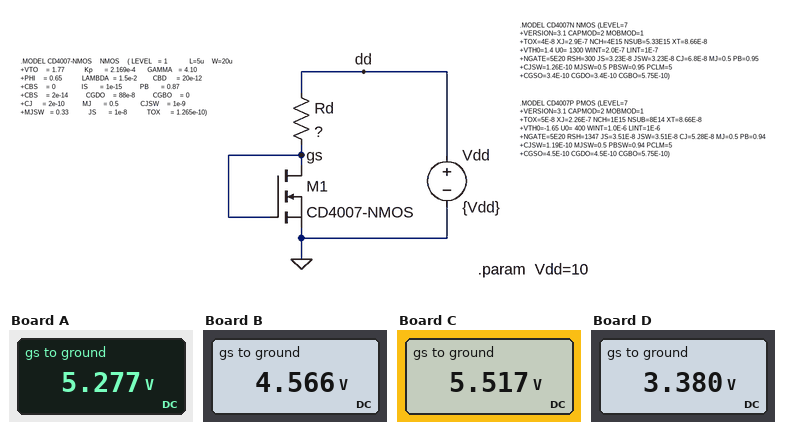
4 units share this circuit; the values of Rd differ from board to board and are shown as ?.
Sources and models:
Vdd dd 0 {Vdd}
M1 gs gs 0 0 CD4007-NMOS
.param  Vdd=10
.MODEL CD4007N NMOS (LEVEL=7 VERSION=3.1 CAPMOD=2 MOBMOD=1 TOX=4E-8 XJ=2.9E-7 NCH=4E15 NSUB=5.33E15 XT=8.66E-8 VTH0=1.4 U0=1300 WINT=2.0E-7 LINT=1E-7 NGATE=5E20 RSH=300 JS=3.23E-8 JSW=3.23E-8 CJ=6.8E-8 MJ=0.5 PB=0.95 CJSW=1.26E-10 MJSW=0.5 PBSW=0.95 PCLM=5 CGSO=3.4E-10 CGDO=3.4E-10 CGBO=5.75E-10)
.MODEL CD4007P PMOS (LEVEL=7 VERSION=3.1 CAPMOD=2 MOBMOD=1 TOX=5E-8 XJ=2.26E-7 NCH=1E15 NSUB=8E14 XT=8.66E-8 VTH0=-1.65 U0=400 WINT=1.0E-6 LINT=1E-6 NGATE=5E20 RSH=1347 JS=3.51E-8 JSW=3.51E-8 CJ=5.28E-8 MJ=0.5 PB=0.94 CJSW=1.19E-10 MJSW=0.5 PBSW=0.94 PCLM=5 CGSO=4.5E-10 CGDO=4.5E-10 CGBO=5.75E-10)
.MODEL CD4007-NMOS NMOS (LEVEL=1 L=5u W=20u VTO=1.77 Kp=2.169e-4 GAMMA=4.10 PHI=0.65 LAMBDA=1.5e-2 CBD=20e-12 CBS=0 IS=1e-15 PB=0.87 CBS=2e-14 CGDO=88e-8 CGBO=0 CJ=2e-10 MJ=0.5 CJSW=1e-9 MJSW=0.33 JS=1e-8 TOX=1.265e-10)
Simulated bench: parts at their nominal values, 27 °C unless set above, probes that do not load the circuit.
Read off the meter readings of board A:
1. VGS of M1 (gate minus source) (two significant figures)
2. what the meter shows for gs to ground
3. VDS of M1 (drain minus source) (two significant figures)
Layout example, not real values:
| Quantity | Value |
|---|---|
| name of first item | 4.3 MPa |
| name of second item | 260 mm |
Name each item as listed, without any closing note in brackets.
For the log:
| Quantity | Value |
|---|---|
| VGS of M1 (gate minus source) | 5.3 V |
| what the meter shows for gs to ground | 5.277 V |
| VDS of M1 (drain minus source) | 5.3 V |
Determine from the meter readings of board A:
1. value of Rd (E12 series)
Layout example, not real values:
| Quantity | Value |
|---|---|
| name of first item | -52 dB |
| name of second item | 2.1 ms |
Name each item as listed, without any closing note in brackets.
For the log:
| Quantity | Value |
|---|---|
| value of Rd | 820 Ω |
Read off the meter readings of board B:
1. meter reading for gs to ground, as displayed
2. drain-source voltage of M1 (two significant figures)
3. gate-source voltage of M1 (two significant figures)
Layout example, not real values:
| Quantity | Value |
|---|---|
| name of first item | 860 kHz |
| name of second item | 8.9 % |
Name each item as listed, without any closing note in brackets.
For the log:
| Quantity | Value |
|---|---|
| meter reading for gs to ground, as displayed | 4.566 V |
| drain-source voltage of M1 | 4.6 V |
| gate-source voltage of M1 | 4.6 V |
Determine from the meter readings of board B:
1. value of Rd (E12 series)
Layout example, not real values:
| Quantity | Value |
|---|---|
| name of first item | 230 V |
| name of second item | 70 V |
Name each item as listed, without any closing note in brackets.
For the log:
| Quantity | Value |
|---|---|
| value of Rd | 1.5 kΩ |
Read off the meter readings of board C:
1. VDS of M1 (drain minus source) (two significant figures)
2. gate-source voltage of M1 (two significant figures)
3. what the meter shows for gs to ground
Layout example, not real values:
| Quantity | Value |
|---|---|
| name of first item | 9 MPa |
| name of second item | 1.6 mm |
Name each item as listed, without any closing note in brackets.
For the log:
| Quantity | Value |
|---|---|
| VDS of M1 (drain minus source) | 5.5 V |
| gate-source voltage of M1 | 5.5 V |
| what the meter shows for gs to ground | 5.517 V |
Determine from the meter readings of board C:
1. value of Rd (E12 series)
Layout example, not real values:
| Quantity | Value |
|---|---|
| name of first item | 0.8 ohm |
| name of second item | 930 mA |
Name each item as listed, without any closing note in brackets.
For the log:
| Quantity | Value |
|---|---|
| value of Rd | 680 Ω |
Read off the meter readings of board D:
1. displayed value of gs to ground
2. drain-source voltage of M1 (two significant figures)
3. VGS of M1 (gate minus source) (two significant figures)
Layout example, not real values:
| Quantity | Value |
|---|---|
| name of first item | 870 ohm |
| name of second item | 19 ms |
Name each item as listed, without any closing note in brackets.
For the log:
| Quantity | Value |
|---|---|
| displayed value of gs to ground | 3.380 V |
| drain-source voltage of M1 | 3.4 V |
| VGS of M1 (gate minus source) | 3.4 V |
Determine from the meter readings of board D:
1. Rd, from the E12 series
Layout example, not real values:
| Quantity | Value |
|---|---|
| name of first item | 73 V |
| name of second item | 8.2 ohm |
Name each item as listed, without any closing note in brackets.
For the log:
| Quantity | Value |
|---|---|
| Rd, from the E12 series | 5.6 kΩ |
